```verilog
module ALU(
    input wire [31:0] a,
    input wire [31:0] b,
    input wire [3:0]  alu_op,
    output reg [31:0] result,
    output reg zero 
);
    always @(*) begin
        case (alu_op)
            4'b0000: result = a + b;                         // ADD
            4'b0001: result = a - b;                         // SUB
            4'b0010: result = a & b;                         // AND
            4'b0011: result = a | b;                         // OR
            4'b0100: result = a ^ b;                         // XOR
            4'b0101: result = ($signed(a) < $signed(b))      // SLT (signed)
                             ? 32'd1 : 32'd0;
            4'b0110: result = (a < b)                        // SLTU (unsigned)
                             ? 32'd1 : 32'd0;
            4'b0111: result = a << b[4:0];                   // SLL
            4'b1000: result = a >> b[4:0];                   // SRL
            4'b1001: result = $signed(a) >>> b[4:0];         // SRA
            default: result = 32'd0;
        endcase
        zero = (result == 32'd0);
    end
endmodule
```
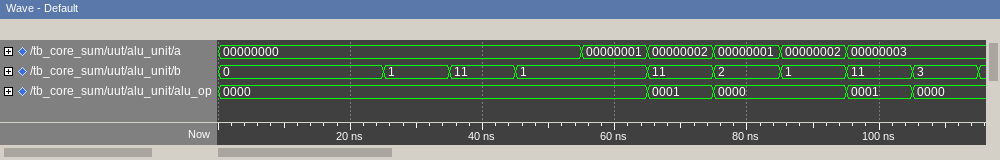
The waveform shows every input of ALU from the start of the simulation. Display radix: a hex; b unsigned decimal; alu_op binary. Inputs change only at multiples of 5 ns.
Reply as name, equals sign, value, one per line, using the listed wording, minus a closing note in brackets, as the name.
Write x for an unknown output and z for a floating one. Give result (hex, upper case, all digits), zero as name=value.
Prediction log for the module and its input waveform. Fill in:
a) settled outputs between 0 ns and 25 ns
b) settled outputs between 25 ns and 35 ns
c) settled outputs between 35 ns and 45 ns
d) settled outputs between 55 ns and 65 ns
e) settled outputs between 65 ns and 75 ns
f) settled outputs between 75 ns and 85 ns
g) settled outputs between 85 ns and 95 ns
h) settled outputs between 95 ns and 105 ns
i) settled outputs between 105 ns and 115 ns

settled outputs between 0 ns and 25 ns = result=00000000, zero=1
settled outputs between 25 ns and 35 ns = result=00000001, zero=0
settled outputs between 35 ns and 45 ns = result=0000000B, zero=0
settled outputs between 55 ns and 65 ns = result=00000002, zero=0
settled outputs between 65 ns and 75 ns = result=FFFFFFF7, zero=0
settled outputs between 75 ns and 85 ns = result=00000003, zero=0
settled outputs between 85 ns and 95 ns = result=00000003, zero=0
settled outputs between 95 ns and 105 ns = result=FFFFFFF8, zero=0
settled outputs between 105 ns and 115 ns = result=00000006, zero=0
